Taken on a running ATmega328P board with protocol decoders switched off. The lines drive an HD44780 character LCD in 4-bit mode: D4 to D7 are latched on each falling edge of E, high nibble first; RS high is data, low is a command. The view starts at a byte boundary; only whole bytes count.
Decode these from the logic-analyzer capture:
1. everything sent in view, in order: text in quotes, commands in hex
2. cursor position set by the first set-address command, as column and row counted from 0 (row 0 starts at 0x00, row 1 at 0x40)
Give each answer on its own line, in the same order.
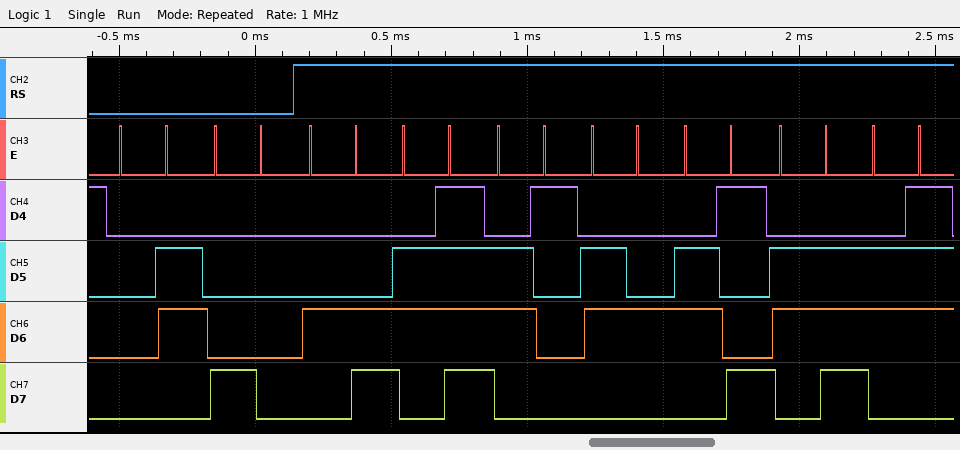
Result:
0x06 0x80 "Loading"
column 0, row 0
